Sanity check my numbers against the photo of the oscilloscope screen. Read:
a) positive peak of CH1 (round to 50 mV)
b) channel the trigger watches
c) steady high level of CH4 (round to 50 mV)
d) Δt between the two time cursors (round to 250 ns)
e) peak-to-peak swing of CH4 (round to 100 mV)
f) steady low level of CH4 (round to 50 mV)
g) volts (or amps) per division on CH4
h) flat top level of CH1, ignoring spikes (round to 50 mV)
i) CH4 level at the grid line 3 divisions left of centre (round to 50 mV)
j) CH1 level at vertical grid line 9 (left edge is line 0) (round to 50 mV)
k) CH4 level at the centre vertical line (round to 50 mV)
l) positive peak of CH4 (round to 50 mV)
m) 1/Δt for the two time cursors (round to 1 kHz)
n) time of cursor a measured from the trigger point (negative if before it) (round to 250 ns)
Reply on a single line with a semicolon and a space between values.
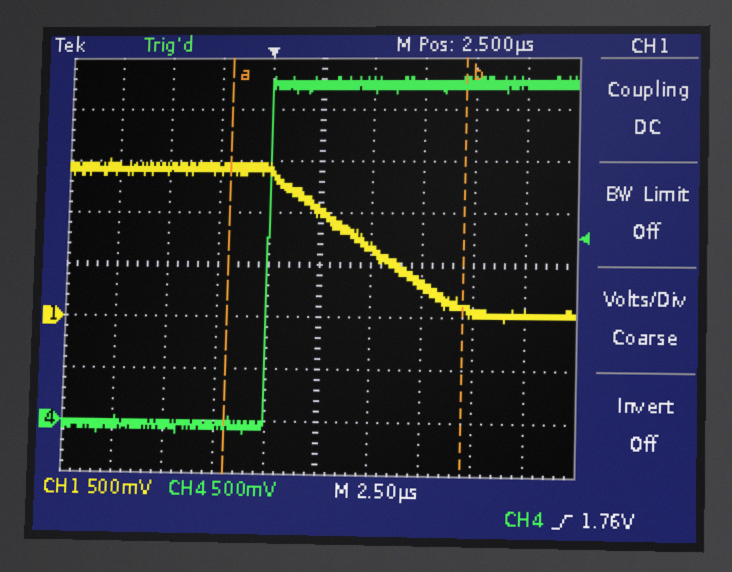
1.50 V; CH4; 3.25 V; 11.50 µs; 3.40 V; -50 mV; 500 mV; 1.45 V; -50 mV; 50 mV; 3.25 V; 3.30 V; 87 kHz; -2.00 µs
